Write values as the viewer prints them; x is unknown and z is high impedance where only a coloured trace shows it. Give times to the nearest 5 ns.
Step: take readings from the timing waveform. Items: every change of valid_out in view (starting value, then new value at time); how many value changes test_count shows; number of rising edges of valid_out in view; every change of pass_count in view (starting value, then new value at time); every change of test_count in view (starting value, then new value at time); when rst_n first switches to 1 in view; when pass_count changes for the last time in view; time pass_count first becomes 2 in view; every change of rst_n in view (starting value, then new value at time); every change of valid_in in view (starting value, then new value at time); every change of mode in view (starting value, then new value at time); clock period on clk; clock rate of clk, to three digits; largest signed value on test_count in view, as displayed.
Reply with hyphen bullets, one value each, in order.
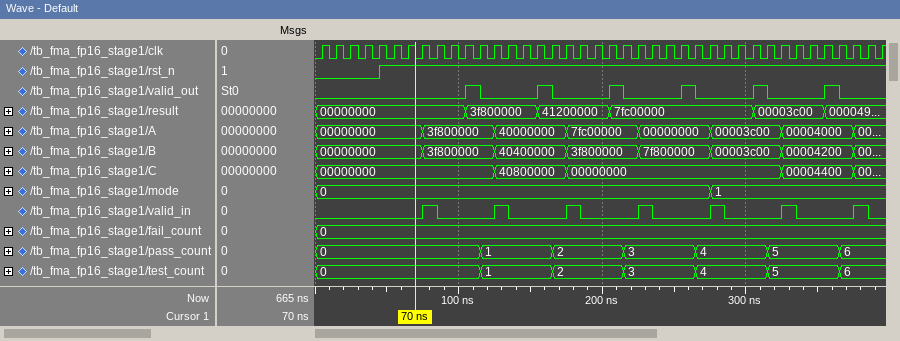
- 0, 1 at 105 ns, 0 at 115 ns, 1 at 155 ns, 0 at 165 ns, 1 at 205 ns, 0 at 215 ns, 1 at 255 ns, 0 at 265 ns, 1 at 305 ns, 0 at 315 ns, 1 at 355 ns, 0 at 365 ns
- 6
- 6
- 0, 1 at 115 ns, 2 at 165 ns, 3 at 215 ns, 4 at 265 ns, 5 at 315 ns, 6 at 365 ns
- 0, 1 at 115 ns, 2 at 165 ns, 3 at 215 ns, 4 at 265 ns, 5 at 315 ns, 6 at 365 ns
- 45 ns
- 365 ns
- 165 ns
- 0, 1 at 45 ns
- 0, 1 at 75 ns, 0 at 85 ns, 1 at 125 ns, 0 at 135 ns, 1 at 175 ns, 0 at 185 ns, 1 at 225 ns, 0 at 235 ns, 1 at 275 ns, 0 at 285 ns, 1 at 325 ns, 0 at 335 ns, 1 at 375 ns, 0 at 385 ns
- 0, 1 at 275 ns
- 10 ns
- 100 MHz
- 6
